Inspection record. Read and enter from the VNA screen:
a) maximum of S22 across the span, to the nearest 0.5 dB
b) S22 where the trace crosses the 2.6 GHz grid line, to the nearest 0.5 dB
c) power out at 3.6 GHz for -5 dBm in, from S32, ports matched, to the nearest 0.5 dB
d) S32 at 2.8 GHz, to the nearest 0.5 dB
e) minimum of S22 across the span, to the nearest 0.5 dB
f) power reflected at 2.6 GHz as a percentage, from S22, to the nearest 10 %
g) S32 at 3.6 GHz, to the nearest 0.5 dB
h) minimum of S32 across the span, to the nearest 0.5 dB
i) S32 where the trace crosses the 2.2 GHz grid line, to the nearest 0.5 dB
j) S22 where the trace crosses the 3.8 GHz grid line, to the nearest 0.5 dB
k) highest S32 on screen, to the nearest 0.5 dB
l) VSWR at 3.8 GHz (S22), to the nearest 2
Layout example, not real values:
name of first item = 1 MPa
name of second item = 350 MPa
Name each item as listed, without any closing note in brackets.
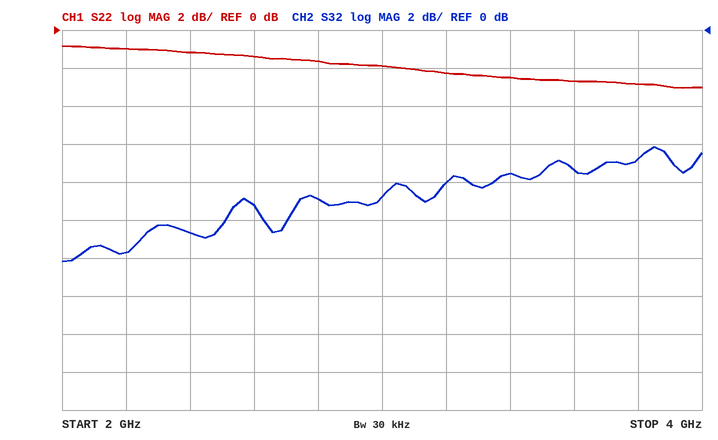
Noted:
maximum of S22 across the span, to the nearest 0.5 dB = -1.0 dB
S22 where the trace crosses the 2.6 GHz grid line, to the nearest 0.5 dB = -1.5 dB
power out at 3.6 GHz for -5 dBm in, from S32, ports matched, to the nearest 0.5 dB = -12.5 dBm
S32 at 2.8 GHz, to the nearest 0.5 dB = -9.0 dB
minimum of S22 across the span, to the nearest 0.5 dB = -3.0 dB
power reflected at 2.6 GHz as a percentage, from S22, to the nearest 10 % = 70 %
S32 at 3.6 GHz, to the nearest 0.5 dB = -7.5 dB
minimum of S32 across the span, to the nearest 0.5 dB = -12.0 dB
S32 where the trace crosses the 2.2 GHz grid line, to the nearest 0.5 dB = -11.5 dB
S22 where the trace crosses the 3.8 GHz grid line, to the nearest 0.5 dB = -3.0 dB
highest S32 on screen, to the nearest 0.5 dB = -6.0 dB
VSWR at 3.8 GHz (S22), to the nearest 2 = 6
